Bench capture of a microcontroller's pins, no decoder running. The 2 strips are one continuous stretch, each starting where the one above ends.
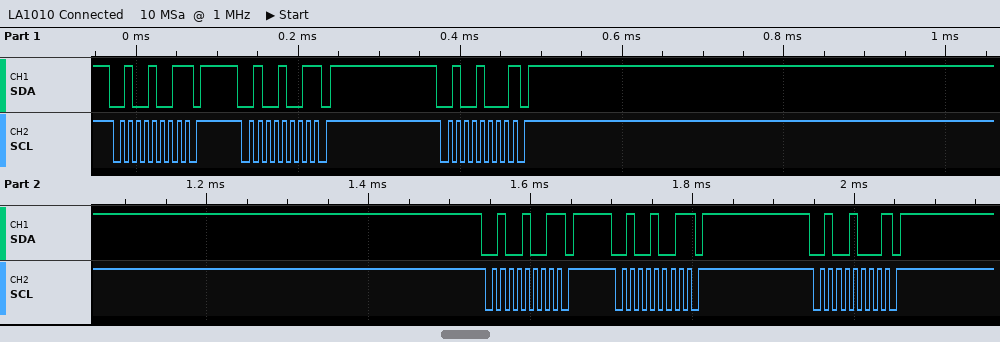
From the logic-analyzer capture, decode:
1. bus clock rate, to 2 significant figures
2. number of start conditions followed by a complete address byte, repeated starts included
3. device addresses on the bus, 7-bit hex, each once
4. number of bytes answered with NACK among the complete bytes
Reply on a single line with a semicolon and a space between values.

100 kHz; 6; 0x24; 6
